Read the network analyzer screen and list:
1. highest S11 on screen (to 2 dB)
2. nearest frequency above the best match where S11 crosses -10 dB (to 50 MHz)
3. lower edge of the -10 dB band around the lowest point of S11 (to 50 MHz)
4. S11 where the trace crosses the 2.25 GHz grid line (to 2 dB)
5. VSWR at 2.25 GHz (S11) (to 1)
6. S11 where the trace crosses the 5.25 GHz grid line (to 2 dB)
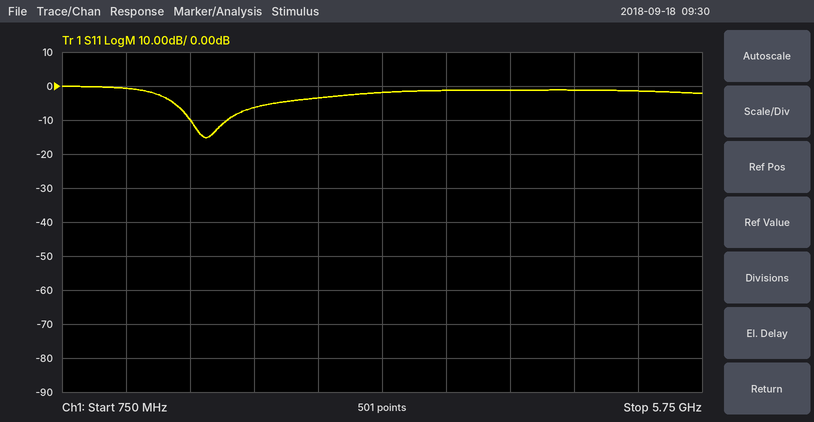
0 dB
2.05 GHz
1.75 GHz
-6 dB
3
-2 dB
